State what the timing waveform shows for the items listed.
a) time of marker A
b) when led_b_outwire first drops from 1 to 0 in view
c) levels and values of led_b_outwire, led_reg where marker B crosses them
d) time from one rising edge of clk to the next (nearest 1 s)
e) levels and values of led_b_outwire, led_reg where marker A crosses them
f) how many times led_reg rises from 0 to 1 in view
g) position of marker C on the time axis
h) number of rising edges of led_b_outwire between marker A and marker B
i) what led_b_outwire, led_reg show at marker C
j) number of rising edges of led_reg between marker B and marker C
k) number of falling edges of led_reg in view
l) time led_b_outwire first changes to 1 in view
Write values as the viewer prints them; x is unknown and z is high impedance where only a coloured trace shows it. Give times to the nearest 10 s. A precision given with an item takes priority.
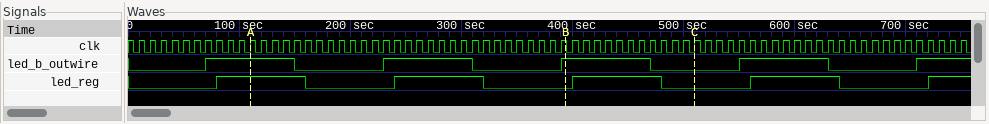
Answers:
110 s
150 s
led_b_outwire=1, led_reg=0
10 s
led_b_outwire=1, led_reg=1
5
510 s
2
led_b_outwire=0, led_reg=0
1
4
70 s
